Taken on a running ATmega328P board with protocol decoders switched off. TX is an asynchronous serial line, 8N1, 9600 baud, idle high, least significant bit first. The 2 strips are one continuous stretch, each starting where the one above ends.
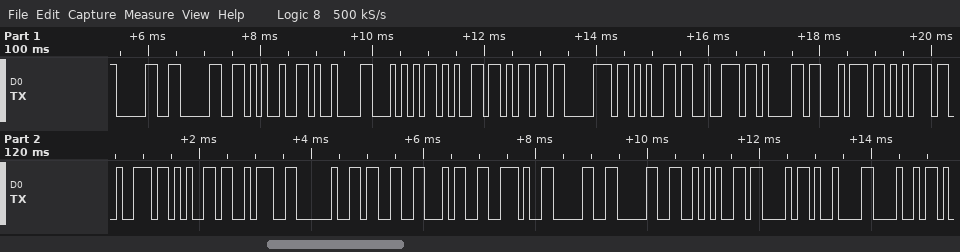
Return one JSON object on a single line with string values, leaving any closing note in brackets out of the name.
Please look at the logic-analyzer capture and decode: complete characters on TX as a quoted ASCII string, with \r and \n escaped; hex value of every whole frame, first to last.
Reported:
{"complete characters on TX as a quoted ASCII string, with \\r and \\n escaped": "\"00%\\tTemperature: 34.00*C\\tH\"", "hex value of every whole frame, first to last": "30 30 25 09 54 65 6D 70 65 72 61 74 75 72 65 3A 20 33 34 2E 30 30 2A 43 09 48"}
